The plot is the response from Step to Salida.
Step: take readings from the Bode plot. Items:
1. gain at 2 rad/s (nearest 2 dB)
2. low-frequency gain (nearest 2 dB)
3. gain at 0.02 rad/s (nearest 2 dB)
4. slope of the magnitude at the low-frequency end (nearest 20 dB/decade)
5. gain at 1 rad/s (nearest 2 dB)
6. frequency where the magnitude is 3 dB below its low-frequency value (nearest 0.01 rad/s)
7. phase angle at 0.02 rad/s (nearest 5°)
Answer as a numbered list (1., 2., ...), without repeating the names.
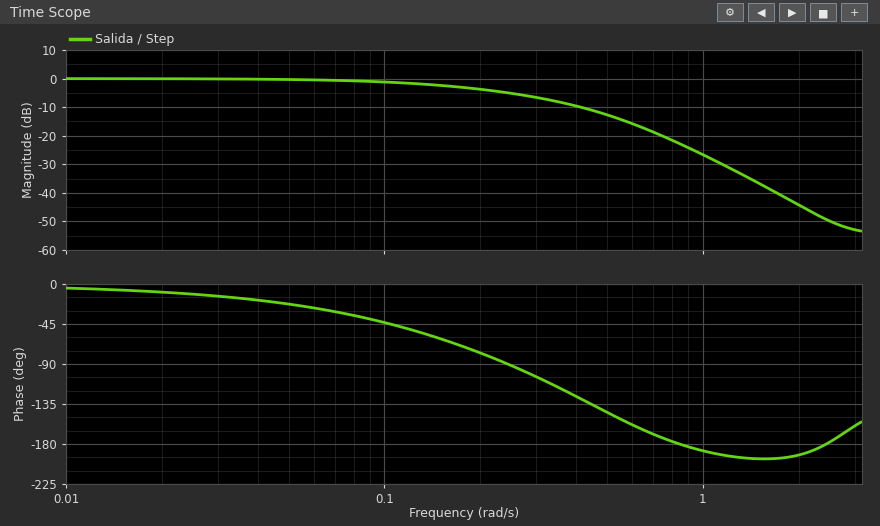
1. -44 dB
2. 0 dB
3. 0 dB
4. 0 dB/decade
5. -26 dB
6. 0.17 rad/s
7. -10°
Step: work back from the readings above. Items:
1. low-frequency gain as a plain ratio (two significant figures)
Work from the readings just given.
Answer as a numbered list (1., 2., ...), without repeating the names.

1. 1.0
